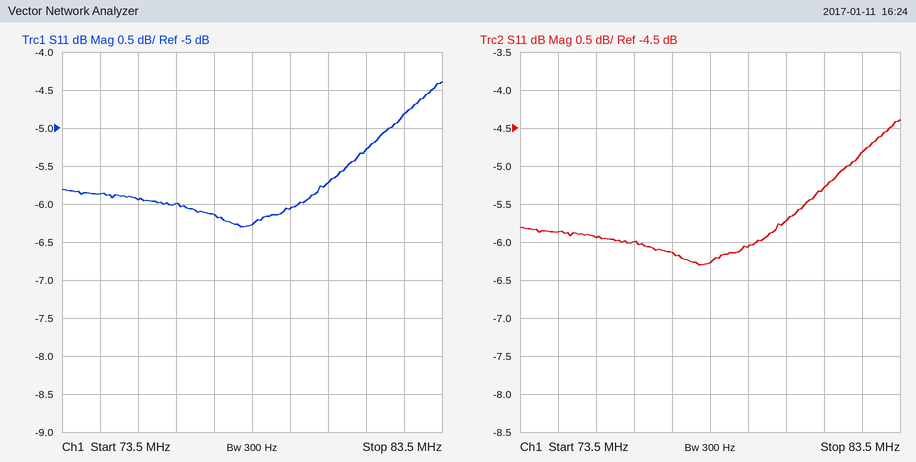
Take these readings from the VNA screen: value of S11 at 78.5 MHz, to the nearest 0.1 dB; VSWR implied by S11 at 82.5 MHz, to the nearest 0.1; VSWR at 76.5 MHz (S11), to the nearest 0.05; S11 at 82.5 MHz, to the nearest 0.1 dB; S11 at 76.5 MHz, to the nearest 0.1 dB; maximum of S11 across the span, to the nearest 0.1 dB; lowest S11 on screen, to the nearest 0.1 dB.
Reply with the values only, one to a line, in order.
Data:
-6.3 dB
3.7
3.00
-4.8 dB
-6.0 dB
-4.4 dB
-6.3 dB
